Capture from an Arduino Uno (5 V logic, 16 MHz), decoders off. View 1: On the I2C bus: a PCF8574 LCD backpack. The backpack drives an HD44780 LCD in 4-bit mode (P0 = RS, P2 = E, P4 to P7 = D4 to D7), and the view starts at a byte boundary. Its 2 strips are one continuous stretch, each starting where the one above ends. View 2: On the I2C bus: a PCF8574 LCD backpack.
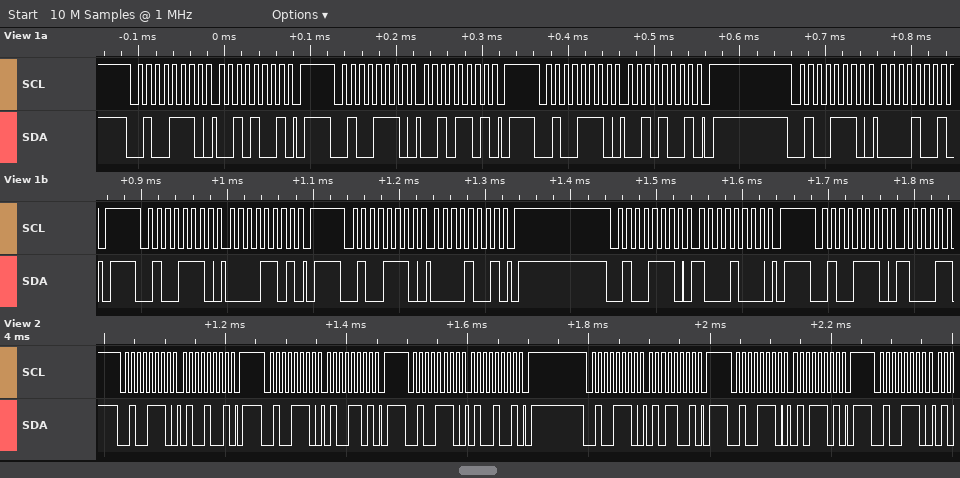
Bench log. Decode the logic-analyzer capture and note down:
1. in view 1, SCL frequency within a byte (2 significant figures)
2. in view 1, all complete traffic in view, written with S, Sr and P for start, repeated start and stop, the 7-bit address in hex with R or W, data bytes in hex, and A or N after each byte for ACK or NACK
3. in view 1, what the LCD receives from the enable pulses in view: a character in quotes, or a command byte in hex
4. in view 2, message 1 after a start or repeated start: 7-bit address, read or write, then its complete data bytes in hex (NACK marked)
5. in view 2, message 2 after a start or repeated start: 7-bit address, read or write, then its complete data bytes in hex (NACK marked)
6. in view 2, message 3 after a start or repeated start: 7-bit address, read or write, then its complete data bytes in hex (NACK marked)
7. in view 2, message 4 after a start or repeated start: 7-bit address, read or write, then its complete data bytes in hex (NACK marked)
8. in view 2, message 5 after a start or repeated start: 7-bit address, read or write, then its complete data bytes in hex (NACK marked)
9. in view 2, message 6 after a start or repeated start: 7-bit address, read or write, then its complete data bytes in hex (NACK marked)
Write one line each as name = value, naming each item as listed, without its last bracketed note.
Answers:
in view 1, SCL frequency within a byte = 100 kHz
in view 1, all complete traffic in view, written with S, Sr and P for start, repeated start and stop, the 7-bit address in hex with R or W, data bytes in hex, and A or N after each byte for ACK or NACK = S 27W A 29 A P S 27W A 2D A P S 27W A 29 A P S 27W A 09 A P S 27W A 0D A P S 27W A 09 A P S 27W A 88 A P S 27W A
in view 1, what the LCD receives from the enable pulses in view: a character in quotes, or a command byte in hex = ' '
in view 2, message 1 after a start or repeated start: 7-bit address, read or write, then its complete data bytes in hex = 0x27 write: 49
in view 2, message 2 after a start or repeated start: 7-bit address, read or write, then its complete data bytes in hex = 0x27 write: 4D
in view 2, message 3 after a start or repeated start: 7-bit address, read or write, then its complete data bytes in hex = 0x27 write: 49
in view 2, message 4 after a start or repeated start: 7-bit address, read or write, then its complete data bytes in hex = 0x27 write: 59
in view 2, message 5 after a start or repeated start: 7-bit address, read or write, then its complete data bytes in hex = 0x27 write: 5D
in view 2, message 6 after a start or repeated start: 7-bit address, read or write, then its complete data bytes in hex = 0x27 write
